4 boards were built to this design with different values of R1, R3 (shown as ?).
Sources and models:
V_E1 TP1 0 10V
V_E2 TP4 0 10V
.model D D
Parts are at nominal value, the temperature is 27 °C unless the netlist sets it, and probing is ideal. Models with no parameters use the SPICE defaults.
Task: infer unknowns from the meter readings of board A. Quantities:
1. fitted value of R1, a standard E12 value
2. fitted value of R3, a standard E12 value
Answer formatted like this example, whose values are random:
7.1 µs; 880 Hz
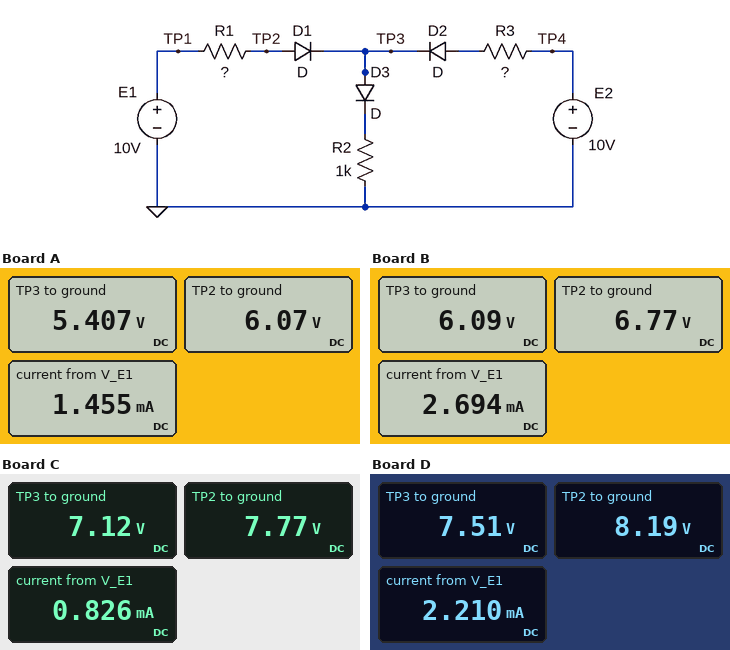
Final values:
2.7 kΩ; 1.2 kΩ
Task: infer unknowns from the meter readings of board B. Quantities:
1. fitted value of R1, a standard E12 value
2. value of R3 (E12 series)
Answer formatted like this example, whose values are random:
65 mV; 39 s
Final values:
1.2 kΩ; 1.2 kΩ
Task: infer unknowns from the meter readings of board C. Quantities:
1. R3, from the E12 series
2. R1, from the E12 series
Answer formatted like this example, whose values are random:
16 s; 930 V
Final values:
390 Ω; 2.7 kΩ
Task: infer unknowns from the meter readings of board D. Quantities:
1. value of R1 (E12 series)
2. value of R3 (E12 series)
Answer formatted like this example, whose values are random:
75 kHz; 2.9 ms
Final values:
820 Ω; 390 Ω
